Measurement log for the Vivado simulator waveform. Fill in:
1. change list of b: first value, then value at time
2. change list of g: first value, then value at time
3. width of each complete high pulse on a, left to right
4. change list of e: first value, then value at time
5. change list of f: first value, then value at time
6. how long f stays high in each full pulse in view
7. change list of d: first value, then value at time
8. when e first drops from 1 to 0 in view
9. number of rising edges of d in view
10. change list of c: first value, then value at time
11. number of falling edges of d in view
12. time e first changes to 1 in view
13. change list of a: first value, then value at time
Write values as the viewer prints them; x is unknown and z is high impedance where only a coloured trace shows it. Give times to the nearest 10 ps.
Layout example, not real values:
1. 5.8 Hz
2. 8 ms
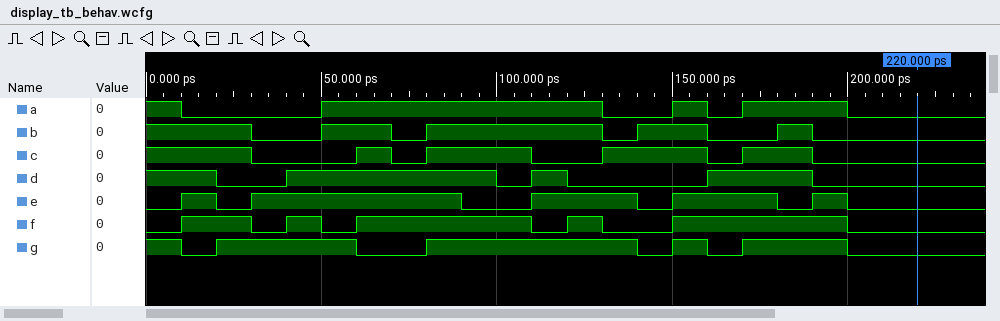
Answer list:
1. 1, 0 at 30 ps, 1 at 50 ps, 0 at 70 ps, 1 at 80 ps, 0 at 130 ps, 1 at 140 ps, 0 at 160 ps, 1 at 180 ps, 0 at 190 ps
2. 1, 0 at 10 ps, 1 at 20 ps, 0 at 60 ps, 1 at 80 ps, 0 at 140 ps, 1 at 150 ps, 0 at 160 ps, 1 at 170 ps, 0 at 200 ps
3. 80 ps, 10 ps, 30 ps
4. 0, 1 at 10 ps, 0 at 20 ps, 1 at 30 ps, 0 at 90 ps, 1 at 110 ps, 0 at 140 ps, 1 at 150 ps, 0 at 180 ps, 1 at 190 ps, 0 at 200 ps
5. 0, 1 at 10 ps, 0 at 30 ps, 1 at 40 ps, 0 at 50 ps, 1 at 60 ps, 0 at 110 ps, 1 at 120 ps, 0 at 130 ps, 1 at 150 ps, 0 at 200 ps
6. 20 ps, 10 ps, 50 ps, 10 ps, 50 ps
7. 1, 0 at 20 ps, 1 at 40 ps, 0 at 100 ps, 1 at 110 ps, 0 at 120 ps, 1 at 160 ps, 0 at 190 ps
8. 20 ps
9. 3
10. 1, 0 at 30 ps, 1 at 60 ps, 0 at 70 ps, 1 at 80 ps, 0 at 110 ps, 1 at 130 ps, 0 at 160 ps, 1 at 170 ps, 0 at 190 ps
11. 4
12. 10 ps
13. 1, 0 at 10 ps, 1 at 50 ps, 0 at 130 ps, 1 at 150 ps, 0 at 160 ps, 1 at 170 ps, 0 at 200 ps
